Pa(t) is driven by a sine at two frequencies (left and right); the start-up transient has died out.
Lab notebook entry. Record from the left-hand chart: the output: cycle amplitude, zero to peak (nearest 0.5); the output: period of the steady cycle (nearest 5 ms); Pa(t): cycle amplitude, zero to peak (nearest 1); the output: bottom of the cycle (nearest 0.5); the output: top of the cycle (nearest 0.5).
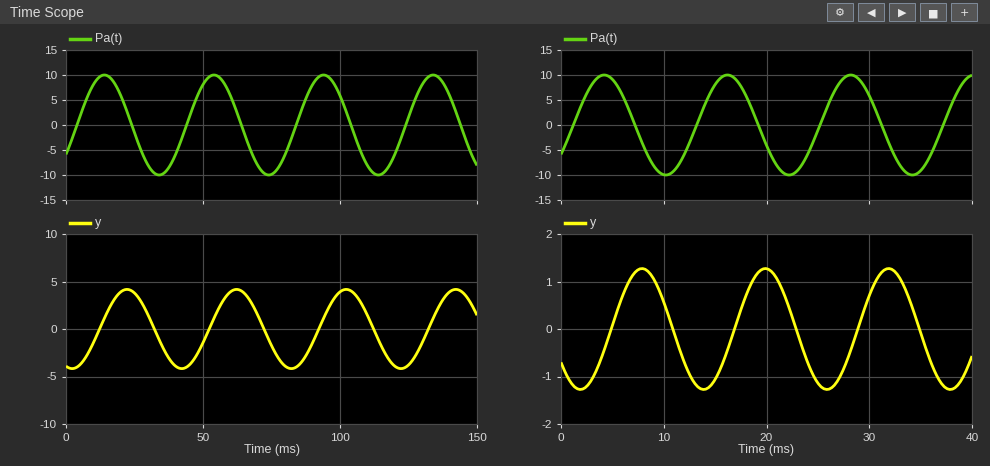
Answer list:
4.0
40 ms
10
-4.0
4.0
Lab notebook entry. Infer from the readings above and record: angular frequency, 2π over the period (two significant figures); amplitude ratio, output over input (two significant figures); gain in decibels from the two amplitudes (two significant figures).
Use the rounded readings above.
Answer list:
0.16 rad/ms
0.40
-8.0 dB
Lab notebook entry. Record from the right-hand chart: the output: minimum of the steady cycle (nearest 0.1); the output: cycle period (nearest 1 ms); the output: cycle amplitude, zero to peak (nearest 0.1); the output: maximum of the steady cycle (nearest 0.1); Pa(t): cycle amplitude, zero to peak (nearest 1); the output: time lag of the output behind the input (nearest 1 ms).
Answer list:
-1.3
12 ms
1.3
1.3
10
4 ms
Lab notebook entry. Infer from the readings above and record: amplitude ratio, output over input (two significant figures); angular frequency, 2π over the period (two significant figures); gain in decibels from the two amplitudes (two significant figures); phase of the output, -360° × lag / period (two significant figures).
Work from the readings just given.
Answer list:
0.13
0.52 rad/ms
-18 dB
-120°
